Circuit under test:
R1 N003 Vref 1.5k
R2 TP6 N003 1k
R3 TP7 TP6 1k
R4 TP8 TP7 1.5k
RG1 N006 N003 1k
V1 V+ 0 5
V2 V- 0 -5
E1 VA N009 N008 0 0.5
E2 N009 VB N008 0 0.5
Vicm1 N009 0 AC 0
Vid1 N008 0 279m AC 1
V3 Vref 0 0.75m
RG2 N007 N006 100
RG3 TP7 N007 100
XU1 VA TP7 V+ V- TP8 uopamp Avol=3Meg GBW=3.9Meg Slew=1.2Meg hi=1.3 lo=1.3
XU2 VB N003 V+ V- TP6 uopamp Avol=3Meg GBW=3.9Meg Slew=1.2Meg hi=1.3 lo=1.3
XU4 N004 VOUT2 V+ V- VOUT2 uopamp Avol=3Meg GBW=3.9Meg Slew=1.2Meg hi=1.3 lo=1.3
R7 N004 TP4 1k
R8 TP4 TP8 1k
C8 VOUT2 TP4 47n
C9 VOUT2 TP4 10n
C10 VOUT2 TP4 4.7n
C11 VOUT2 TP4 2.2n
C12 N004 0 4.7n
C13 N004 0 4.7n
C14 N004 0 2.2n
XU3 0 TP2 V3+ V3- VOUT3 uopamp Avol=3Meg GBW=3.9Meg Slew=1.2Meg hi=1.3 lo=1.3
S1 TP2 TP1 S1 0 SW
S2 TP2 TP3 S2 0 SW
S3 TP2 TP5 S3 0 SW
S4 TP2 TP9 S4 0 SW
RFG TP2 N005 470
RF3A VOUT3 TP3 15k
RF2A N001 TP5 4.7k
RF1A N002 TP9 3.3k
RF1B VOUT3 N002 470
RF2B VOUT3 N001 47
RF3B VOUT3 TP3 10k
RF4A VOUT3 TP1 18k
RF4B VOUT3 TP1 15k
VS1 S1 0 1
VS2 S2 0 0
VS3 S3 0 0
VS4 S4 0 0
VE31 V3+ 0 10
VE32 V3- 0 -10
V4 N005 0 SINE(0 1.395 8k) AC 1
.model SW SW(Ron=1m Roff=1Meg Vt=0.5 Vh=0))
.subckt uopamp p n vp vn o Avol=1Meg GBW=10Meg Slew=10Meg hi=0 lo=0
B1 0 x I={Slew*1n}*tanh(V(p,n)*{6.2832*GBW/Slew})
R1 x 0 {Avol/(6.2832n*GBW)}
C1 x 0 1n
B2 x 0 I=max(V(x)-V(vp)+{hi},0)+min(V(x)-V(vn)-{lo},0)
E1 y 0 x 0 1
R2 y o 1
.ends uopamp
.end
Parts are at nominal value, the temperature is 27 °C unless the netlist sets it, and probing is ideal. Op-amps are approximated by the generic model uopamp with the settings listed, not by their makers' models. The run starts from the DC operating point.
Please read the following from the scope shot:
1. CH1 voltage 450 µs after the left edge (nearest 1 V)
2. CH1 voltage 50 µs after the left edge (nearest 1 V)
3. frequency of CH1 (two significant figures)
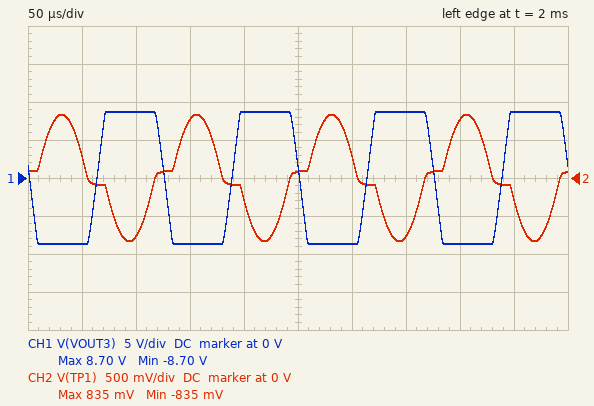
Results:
9 V
-9 V
8.0 kHz
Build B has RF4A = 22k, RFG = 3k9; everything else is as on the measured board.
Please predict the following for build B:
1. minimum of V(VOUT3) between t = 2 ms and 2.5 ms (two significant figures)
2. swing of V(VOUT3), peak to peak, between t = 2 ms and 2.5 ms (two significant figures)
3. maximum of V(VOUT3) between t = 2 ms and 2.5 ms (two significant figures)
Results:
-3.1 V
6.2 V
3.1 V
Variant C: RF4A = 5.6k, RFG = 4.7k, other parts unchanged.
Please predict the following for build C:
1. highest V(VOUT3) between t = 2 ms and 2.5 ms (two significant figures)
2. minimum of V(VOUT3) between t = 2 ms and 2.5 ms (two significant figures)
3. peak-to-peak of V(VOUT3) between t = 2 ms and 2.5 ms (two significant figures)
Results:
1.2 V
-1.2 V
2.4 V
